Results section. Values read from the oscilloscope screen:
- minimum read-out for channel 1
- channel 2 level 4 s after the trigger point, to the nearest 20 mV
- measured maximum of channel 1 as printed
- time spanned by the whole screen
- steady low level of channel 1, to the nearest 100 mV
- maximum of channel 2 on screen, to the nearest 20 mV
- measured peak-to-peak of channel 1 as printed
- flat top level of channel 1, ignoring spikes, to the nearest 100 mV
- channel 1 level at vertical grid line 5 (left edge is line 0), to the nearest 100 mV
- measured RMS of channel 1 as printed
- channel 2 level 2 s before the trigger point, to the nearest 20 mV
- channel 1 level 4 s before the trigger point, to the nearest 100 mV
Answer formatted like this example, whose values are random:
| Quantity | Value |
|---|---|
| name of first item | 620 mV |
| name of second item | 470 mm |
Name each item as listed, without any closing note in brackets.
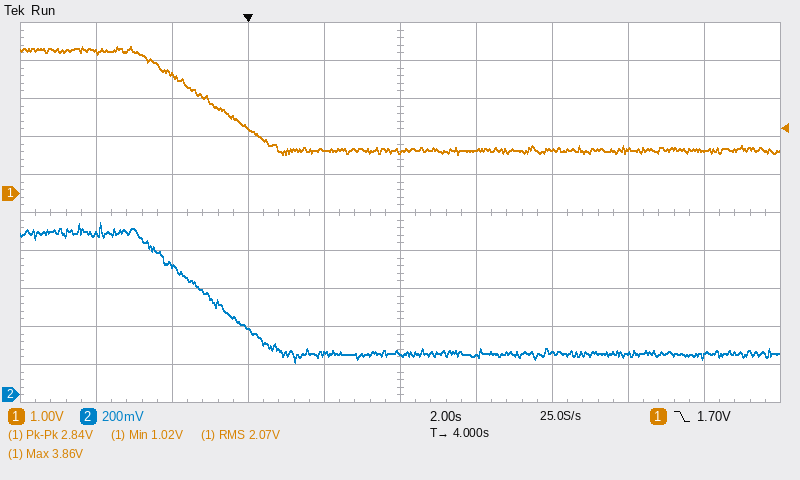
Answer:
| Quantity | Value |
|---|---|
| minimum read-out for channel 1 | 1.02 V |
| channel 2 level 4 s after the trigger point, to the nearest 20 mV | 220 mV |
| measured maximum of channel 1 as printed | 3.86 V |
| time spanned by the whole screen | 20 s |
| steady low level of channel 1, to the nearest 100 mV | 1.1 V |
| maximum of channel 2 on screen, to the nearest 20 mV | 900 mV |
| measured peak-to-peak of channel 1 as printed | 2.84 V |
| flat top level of channel 1, ignoring spikes, to the nearest 100 mV | 3.8 V |
| channel 1 level at vertical grid line 5 (left edge is line 0), to the nearest 100 mV | 1.1 V |
| measured RMS of channel 1 as printed | 2.07 V |
| channel 2 level 2 s before the trigger point, to the nearest 20 mV | 680 mV |
| channel 1 level 4 s before the trigger point, to the nearest 100 mV | 3.7 V |
